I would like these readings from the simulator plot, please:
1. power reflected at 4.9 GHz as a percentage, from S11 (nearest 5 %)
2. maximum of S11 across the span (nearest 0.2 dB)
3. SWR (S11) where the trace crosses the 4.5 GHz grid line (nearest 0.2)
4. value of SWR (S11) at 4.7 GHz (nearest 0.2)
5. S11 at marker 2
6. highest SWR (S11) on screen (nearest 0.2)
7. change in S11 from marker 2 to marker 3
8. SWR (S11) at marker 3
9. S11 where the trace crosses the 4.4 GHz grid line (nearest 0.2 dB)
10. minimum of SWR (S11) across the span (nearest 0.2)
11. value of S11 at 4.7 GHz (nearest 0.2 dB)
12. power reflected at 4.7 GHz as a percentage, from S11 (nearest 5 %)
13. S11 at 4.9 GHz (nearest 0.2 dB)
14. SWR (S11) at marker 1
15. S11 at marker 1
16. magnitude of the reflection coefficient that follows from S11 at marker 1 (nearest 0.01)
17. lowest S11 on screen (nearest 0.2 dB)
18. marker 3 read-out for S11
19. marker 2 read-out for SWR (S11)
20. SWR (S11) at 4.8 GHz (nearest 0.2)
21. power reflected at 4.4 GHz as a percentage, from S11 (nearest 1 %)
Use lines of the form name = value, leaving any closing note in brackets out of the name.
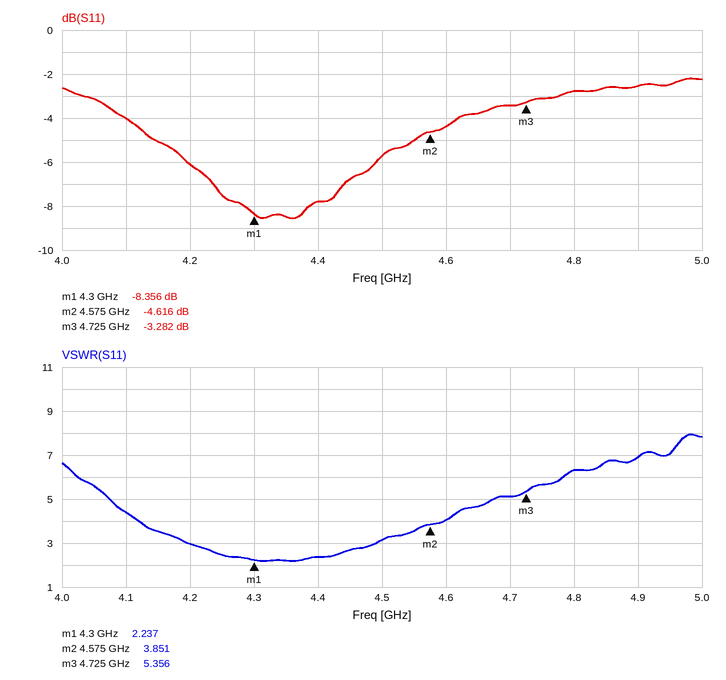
power reflected at 4.9 GHz as a percentage, from S11 = 55 %
maximum of S11 across the span = -2.2 dB
SWR (S11) where the trace crosses the 4.5 GHz grid line = 3.2
value of SWR (S11) at 4.7 GHz = 5.2
S11 at marker 2 = -4.616 dB
highest SWR (S11) on screen = 8.0
change in S11 from marker 2 to marker 3 = 1.334 dB
SWR (S11) at marker 3 = 5.356
S11 where the trace crosses the 4.4 GHz grid line = -7.8 dB
minimum of SWR (S11) across the span = 2.2
value of S11 at 4.7 GHz = -3.4 dB
power reflected at 4.7 GHz as a percentage, from S11 = 45 %
S11 at 4.9 GHz = -2.6 dB
SWR (S11) at marker 1 = 2.237
S11 at marker 1 = -8.356 dB
magnitude of the reflection coefficient that follows from S11 at marker 1 = 0.38
lowest S11 on screen = -8.6 dB
marker 3 read-out for S11 = -3.282 dB
marker 2 read-out for SWR = 3.851
SWR (S11) at 4.8 GHz = 6.4
power reflected at 4.4 GHz as a percentage, from S11 = 17 %
